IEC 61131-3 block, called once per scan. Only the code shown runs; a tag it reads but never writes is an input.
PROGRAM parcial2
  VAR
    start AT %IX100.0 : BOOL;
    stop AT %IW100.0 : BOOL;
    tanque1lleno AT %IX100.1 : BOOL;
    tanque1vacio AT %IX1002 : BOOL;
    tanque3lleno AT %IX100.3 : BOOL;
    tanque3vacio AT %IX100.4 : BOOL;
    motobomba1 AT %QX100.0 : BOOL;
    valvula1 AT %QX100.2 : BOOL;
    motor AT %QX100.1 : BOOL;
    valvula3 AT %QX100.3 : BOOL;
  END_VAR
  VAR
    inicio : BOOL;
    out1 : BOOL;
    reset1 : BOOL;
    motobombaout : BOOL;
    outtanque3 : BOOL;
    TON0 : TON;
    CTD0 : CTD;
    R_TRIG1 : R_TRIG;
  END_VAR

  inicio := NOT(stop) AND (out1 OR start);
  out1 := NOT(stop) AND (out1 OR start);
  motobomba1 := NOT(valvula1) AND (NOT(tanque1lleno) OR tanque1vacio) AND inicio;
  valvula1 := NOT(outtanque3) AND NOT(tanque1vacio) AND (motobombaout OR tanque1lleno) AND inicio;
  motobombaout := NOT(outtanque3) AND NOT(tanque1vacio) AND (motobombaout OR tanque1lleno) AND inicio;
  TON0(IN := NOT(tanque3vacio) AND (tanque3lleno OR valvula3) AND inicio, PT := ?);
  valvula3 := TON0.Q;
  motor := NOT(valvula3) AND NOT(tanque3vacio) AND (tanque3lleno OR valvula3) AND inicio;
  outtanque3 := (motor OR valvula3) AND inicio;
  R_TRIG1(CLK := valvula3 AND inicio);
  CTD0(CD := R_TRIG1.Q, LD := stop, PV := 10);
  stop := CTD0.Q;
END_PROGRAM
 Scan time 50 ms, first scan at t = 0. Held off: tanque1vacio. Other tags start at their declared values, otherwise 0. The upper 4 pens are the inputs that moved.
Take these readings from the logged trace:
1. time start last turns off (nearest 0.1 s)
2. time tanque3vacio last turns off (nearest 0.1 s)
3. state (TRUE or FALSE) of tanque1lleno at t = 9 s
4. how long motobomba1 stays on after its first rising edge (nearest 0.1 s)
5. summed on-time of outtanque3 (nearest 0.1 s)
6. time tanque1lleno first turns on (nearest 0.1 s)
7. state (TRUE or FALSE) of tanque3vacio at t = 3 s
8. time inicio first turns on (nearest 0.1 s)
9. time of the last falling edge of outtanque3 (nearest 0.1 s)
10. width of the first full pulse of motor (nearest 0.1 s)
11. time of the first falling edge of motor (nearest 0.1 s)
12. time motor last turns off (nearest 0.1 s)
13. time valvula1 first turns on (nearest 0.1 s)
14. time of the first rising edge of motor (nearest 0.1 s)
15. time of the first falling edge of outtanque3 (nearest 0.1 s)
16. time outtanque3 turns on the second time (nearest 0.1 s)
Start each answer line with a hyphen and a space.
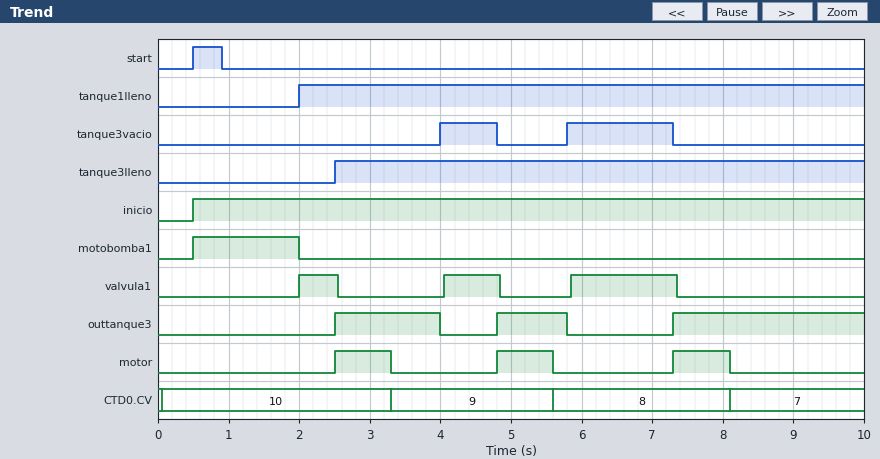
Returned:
- 0.9 s
- 7.3 s
- TRUE
- 1.5 s
- 5.2 s
- 2.0 s
- FALSE
- 0.5 s
- 5.8 s
- 0.8 s
- 3.3 s
- 8.1 s
- 2.0 s
- 2.5 s
- 4.0 s
- 4.8 s
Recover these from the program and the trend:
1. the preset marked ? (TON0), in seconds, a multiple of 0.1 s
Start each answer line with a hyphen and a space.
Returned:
- 0.8 s
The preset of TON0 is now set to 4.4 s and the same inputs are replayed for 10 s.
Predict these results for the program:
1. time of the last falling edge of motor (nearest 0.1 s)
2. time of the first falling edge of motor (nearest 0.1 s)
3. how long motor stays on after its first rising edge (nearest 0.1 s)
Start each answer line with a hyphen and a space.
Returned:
- 5.8 s
- 4.0 s
- 1.5 s
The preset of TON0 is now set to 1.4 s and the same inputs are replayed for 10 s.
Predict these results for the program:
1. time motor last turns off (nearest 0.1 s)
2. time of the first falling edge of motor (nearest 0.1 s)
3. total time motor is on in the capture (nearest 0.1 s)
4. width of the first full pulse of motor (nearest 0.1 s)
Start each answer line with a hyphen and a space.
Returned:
- 8.7 s
- 3.9 s
- 3.8 s
- 1.4 s
